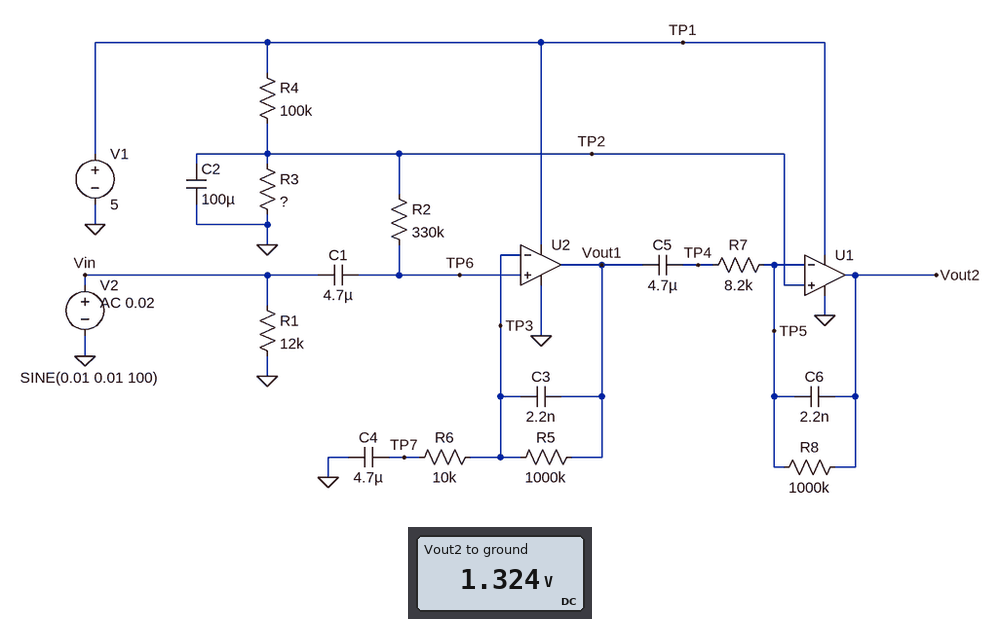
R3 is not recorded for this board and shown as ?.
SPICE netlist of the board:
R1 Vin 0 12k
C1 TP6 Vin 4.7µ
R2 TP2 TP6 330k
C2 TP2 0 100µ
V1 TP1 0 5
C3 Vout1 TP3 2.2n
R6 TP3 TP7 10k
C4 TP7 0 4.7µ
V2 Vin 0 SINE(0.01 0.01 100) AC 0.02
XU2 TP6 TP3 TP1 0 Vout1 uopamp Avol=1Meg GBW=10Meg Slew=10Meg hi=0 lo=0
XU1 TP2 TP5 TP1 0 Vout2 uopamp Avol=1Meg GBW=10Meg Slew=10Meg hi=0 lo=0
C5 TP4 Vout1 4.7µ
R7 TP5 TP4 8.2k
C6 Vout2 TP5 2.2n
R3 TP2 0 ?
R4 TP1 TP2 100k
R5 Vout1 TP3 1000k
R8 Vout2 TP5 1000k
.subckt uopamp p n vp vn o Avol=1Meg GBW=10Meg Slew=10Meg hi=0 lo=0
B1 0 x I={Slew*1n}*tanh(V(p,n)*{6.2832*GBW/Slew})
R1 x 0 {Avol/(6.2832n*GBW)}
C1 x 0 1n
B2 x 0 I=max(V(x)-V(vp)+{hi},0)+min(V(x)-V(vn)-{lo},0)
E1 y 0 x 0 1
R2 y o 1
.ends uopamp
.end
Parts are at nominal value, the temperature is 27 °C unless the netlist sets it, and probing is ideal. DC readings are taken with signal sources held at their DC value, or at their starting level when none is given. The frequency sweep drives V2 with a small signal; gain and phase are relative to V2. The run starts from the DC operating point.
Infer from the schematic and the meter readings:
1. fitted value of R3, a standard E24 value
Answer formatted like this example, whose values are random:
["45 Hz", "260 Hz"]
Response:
["36 kΩ"]
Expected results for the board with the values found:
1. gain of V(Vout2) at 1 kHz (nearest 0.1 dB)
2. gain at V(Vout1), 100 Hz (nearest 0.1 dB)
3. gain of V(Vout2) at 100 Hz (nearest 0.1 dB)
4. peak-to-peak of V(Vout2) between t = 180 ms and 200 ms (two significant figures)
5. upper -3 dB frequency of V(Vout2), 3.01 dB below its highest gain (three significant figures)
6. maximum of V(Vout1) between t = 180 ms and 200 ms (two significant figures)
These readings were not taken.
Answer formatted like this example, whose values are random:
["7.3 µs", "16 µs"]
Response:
["36.2 dB", "35.4 dB", "72.5 dB", "5.0 V", "54.0 Hz", "1.9 V"]
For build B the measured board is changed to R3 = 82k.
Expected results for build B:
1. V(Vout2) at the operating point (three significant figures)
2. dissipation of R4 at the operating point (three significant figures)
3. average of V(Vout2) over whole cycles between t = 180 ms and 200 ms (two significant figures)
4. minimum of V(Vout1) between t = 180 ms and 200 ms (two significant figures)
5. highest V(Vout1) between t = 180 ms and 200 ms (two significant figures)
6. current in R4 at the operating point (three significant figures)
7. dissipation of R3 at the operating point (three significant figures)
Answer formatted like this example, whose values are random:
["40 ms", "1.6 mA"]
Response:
["2.25 V", "75.5 µW", "2.5 V", "1.7 V", "2.8 V", "27.5 µA", "61.9 µW"]
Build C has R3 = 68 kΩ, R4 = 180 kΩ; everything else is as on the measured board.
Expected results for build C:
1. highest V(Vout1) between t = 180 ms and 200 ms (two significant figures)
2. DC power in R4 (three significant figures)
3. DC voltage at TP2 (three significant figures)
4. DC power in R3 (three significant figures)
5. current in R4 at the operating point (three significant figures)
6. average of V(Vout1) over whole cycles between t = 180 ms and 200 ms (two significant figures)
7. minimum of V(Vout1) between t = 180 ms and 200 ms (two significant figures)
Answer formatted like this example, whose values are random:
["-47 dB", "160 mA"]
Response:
["2.0 V", "73.2 µW", "1.37 V", "27.6 µW", "20.2 µA", "1.4 V", "780 mV"]
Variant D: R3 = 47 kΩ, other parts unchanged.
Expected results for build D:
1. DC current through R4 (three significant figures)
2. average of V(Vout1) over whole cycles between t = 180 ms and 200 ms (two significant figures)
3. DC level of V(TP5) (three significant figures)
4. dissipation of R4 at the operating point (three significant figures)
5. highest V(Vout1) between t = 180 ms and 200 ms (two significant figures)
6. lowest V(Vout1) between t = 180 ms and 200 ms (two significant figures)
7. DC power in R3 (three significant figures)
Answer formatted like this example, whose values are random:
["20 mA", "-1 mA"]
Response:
["34.0 µA", "1.6 V", "1.60 V", "116 µW", "2.2 V", "1.0 V", "54.4 µW"]
